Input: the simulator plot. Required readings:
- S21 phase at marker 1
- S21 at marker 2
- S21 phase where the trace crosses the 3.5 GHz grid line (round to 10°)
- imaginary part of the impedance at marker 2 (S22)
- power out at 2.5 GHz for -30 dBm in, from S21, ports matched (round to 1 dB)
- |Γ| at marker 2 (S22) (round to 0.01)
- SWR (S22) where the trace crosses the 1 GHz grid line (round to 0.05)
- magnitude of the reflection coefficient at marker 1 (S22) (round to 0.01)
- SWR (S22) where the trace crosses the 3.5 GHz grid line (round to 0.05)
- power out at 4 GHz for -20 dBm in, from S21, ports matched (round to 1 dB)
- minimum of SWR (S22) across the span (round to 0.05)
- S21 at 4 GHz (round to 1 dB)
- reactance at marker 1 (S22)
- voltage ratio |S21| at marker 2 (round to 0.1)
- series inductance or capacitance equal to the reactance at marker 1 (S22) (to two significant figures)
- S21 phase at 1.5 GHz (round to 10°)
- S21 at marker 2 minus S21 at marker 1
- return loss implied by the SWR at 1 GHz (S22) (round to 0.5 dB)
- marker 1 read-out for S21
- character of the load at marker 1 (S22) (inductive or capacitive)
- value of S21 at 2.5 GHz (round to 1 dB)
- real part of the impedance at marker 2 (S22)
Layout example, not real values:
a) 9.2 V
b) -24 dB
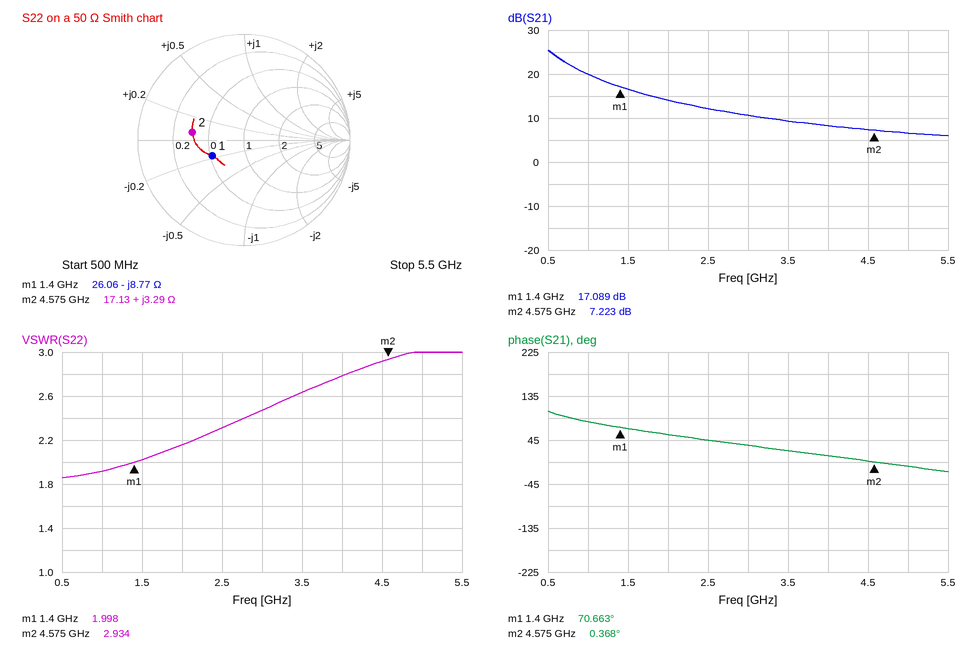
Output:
a) 70.663°
b) 7.223 dB
c) 20°
d) +3.29 Ω
e) -18 dBm
f) 0.49
g) 1.90
h) 0.33
i) 2.65
j) -12 dBm
k) 1.85
l) 8 dB
m) -8.77 Ω
n) 2.3
o) 13 pF
p) 70°
q) -9.866 dB
r) 10.0 dB
s) 17.089 dB
t) capacitive
u) 12 dB
v) 17.13 Ω
